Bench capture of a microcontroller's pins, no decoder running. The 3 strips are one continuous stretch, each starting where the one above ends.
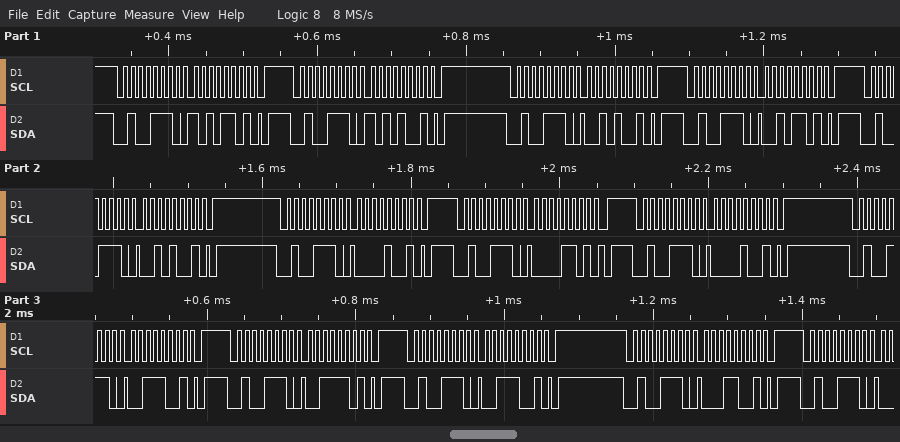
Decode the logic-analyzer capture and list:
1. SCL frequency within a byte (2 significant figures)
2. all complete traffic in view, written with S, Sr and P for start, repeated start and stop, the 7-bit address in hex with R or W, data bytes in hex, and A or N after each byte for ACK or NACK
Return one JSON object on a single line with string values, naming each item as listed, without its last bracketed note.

{"SCL frequency within a byte": "100 kHz", "all complete traffic in view, written with S, Sr and P for start, repeated start and stop, the 7-bit address in hex with R or W, data bytes in hex, and A or N after each byte for ACK or NACK": "S 27W A AD A P S 27W A A9 A P S 27W A 29 A P S 27W A 2D A P S 27W A 29 A P S 27W A 09 A P S 27W A 0D A P S 27W A 09 A P S 27W A 39 A P S 27W A 3D A P S 27W A 39 A P S 27W A 19 A P S 27W A"}
